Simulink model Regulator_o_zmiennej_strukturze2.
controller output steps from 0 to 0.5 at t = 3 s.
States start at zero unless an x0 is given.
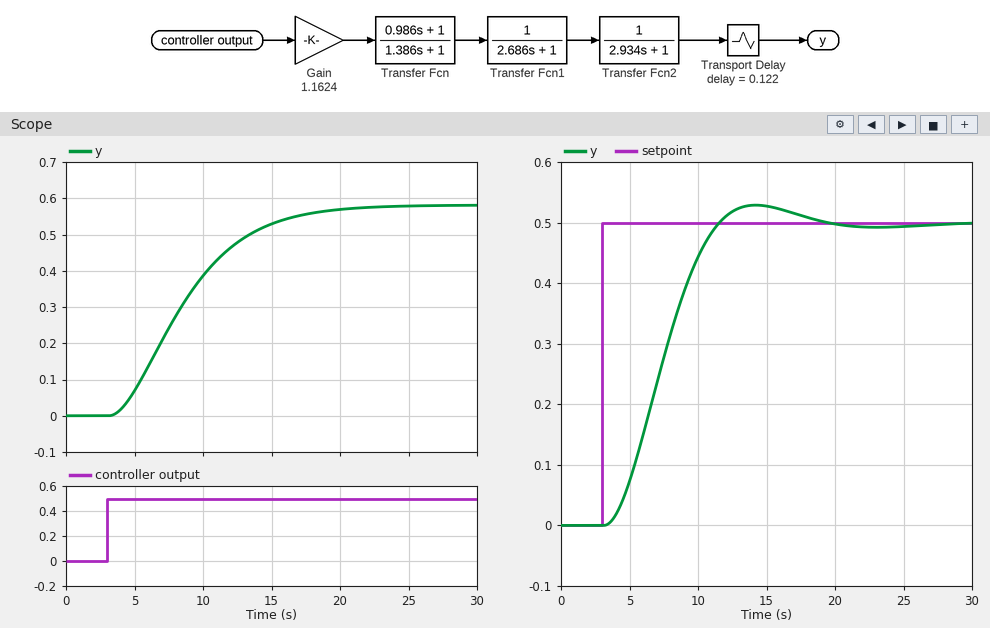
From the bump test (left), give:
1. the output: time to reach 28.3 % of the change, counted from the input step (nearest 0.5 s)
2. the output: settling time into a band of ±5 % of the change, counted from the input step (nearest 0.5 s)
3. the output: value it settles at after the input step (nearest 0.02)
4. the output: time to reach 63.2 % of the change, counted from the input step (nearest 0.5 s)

3.5 s
14.0 s
0.58
6.5 s
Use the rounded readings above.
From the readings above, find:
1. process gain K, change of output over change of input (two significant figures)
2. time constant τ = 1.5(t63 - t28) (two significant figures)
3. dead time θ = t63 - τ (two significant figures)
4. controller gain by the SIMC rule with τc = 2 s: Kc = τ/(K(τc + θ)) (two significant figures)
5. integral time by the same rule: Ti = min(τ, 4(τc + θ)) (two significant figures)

1.2
4.5 s
2.0 s
0.94
4.5 s
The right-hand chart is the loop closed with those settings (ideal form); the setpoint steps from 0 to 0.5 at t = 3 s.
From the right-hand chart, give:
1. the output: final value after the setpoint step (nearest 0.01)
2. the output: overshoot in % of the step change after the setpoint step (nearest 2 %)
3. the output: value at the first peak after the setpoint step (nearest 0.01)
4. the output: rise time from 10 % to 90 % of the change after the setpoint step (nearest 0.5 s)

0.50
6 %
0.53
5.5 s
